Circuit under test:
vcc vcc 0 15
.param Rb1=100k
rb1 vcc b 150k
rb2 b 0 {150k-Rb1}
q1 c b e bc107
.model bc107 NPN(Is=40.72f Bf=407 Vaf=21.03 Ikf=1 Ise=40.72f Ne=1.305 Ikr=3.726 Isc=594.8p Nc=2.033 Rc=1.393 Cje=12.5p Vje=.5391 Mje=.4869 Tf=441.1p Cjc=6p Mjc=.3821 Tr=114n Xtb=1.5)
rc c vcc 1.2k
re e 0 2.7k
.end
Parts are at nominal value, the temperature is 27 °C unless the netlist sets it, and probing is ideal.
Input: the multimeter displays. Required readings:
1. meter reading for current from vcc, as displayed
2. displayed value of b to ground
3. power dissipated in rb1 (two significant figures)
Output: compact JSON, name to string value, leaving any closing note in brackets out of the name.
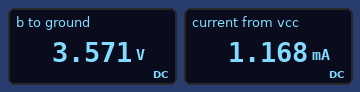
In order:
{"meter reading for current from vcc, as displayed": "1.168 mA", "displayed value of b to ground": "3.571 V", "power dissipated in rb1": "870 µW"}
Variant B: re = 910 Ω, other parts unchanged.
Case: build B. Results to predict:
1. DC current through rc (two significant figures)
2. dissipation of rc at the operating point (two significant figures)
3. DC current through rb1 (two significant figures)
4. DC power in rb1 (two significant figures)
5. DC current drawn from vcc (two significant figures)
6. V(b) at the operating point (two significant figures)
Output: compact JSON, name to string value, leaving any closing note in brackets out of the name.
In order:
{"DC current through rc": "2.9 mA", "dissipation of rc at the operating point": "10 mW", "DC current through rb1": "78 µA", "DC power in rb1": "910 µW", "DC current drawn from vcc": "3.0 mA", "V(b) at the operating point": "3.3 V"}
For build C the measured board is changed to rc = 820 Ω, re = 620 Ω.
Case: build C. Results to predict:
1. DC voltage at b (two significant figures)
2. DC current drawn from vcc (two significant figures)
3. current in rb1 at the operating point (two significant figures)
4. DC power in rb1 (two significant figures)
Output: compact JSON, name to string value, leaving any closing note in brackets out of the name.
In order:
{"DC voltage at b": "3.2 V", "DC current drawn from vcc": "4.1 mA", "current in rb1 at the operating point": "79 µA", "DC power in rb1": "930 µW"}
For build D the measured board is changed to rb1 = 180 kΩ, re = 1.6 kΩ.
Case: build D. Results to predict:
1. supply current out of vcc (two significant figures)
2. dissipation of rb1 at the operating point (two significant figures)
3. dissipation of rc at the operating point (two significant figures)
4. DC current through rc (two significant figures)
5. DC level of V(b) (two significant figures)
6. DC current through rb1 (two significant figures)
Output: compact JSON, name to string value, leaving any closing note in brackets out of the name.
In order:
{"supply current out of vcc": "1.6 mA", "dissipation of rb1 at the operating point": "800 µW", "dissipation of rc at the operating point": "2.7 mW", "DC current through rc": "1.5 mA", "DC level of V(b)": "3.0 V", "DC current through rb1": "67 µA"}
